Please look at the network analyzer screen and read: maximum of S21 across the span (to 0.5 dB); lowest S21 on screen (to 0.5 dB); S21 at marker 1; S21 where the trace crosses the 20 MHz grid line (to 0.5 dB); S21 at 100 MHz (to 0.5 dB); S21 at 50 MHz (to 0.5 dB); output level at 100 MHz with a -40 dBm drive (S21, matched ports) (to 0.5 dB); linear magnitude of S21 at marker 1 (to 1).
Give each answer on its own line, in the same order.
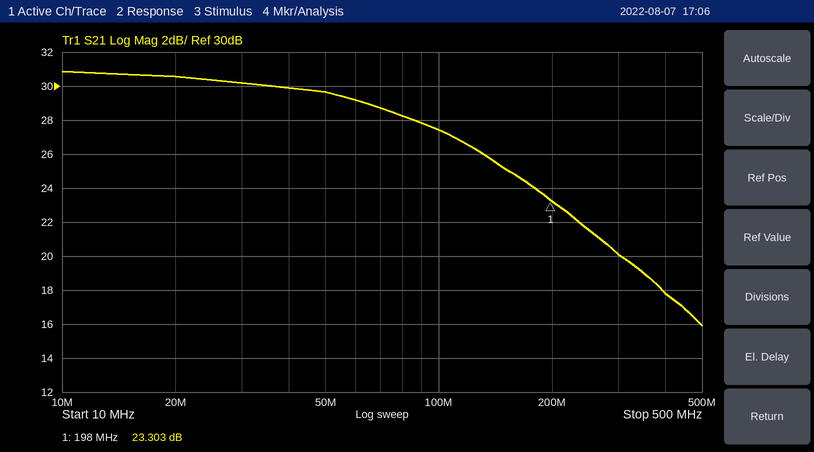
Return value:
31.0 dB
16.0 dB
23.303 dB
30.5 dB
27.5 dB
29.5 dB
-12.5 dBm
15
